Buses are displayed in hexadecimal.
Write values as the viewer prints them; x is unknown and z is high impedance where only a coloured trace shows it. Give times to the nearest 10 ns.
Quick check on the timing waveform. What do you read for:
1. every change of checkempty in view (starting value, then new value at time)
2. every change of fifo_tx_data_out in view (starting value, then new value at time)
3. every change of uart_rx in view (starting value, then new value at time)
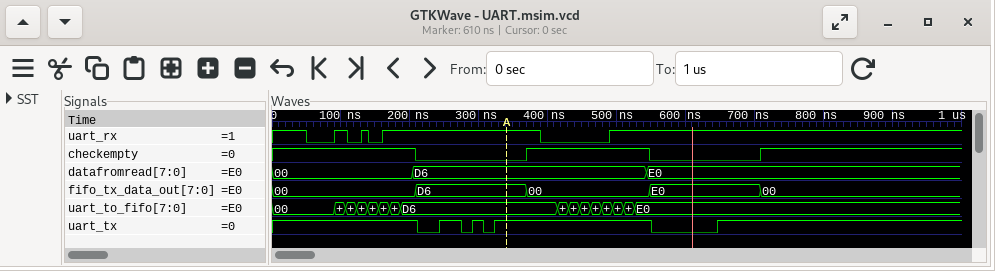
1, 0 at 210 ns, 1 at 370 ns, 0 at 550 ns, 1 at 710 ns
00, D6 at 210 ns, 00 at 370 ns, E0 at 550 ns, 00 at 710 ns
1, 0 at 50 ns, 1 at 90 ns, 0 at 110 ns, 1 at 130 ns, 0 at 140 ns, 1 at 160 ns, 0 at 390 ns, 1 at 490 ns
